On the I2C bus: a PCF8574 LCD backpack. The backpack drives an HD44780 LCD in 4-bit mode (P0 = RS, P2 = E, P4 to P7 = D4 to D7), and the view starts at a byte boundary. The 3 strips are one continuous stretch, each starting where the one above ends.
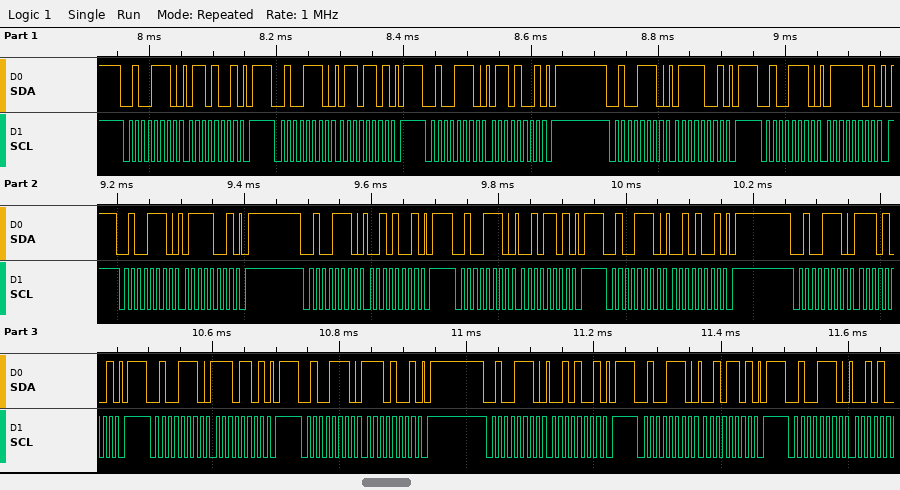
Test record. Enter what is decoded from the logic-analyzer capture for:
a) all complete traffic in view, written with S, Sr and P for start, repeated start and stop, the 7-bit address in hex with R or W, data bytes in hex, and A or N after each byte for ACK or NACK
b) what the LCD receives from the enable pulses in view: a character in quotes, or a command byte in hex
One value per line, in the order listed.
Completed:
S 27W A 69 A P S 27W A 6D A P S 27W A 69 A P S 27W A 79 A P S 27W A 7D A P S 27W A 79 A P S 27W A 29 A P S 27W A 2D A P S 27W A 29 A P S 27W A E9 A P S 27W A ED A P S 27W A E9 A P S 27W A 29 A P S 27W A 2D A P S 27W A
'g' '.'
